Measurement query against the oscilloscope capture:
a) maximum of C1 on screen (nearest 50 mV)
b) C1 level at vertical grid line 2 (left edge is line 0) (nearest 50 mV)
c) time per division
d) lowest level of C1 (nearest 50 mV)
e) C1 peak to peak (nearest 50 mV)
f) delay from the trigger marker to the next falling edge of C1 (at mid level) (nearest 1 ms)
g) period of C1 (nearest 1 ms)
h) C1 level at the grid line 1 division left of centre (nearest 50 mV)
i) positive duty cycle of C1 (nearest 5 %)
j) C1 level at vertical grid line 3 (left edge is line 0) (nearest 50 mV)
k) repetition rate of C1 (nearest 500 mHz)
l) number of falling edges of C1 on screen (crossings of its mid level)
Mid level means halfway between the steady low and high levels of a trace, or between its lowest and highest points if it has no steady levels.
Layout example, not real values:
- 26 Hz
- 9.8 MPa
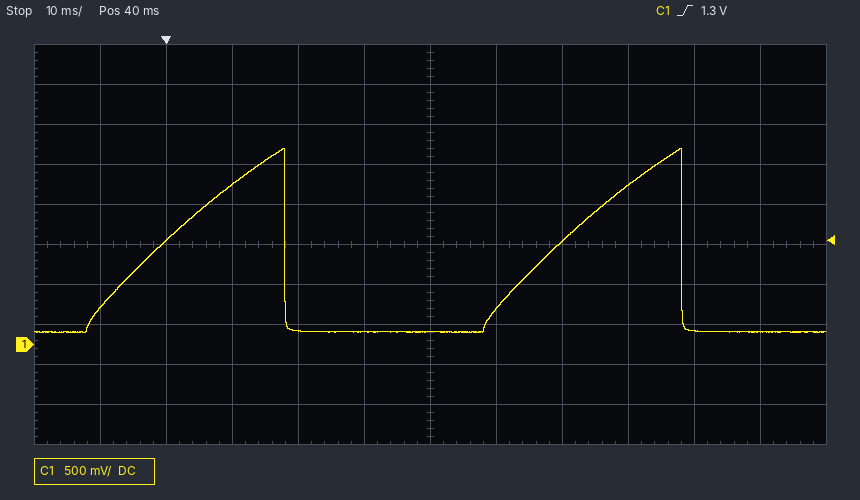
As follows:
- 2.45 V
- 1.30 V
- 10 ms
- 150 mV
- 2.30 V
- 18 ms
- 60 ms
- 150 mV
- 30 %
- 2.00 V
- 16.5 Hz
- 2
